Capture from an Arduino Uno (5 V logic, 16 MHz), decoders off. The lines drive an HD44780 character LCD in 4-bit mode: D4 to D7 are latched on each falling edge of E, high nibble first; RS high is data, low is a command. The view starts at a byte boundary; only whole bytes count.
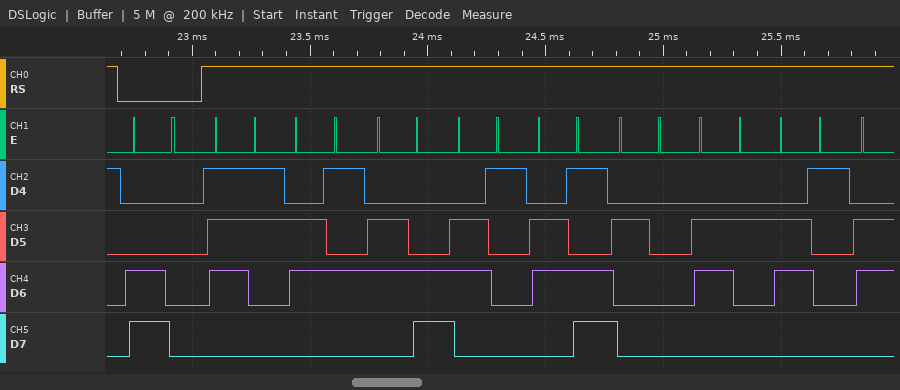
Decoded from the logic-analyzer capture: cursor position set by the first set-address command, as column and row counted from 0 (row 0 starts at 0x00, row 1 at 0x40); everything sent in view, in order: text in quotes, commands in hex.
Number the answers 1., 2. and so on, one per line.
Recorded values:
1. column 0, row 1
2. 0xC0 "selam ba"
